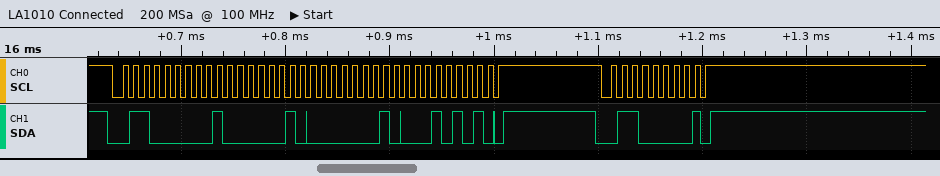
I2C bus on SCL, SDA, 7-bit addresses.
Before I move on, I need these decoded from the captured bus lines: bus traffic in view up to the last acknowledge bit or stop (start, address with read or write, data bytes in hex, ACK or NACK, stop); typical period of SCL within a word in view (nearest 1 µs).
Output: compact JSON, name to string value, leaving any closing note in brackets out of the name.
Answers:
{"bus traffic in view up to the last acknowledge bit or stop": "start, address 30 write ACK, 81 ACK, 01 ACK, 15 ACK, stop, start, address 30 write NACK, stop", "typical period of SCL within a word in view": "10 µs"}
